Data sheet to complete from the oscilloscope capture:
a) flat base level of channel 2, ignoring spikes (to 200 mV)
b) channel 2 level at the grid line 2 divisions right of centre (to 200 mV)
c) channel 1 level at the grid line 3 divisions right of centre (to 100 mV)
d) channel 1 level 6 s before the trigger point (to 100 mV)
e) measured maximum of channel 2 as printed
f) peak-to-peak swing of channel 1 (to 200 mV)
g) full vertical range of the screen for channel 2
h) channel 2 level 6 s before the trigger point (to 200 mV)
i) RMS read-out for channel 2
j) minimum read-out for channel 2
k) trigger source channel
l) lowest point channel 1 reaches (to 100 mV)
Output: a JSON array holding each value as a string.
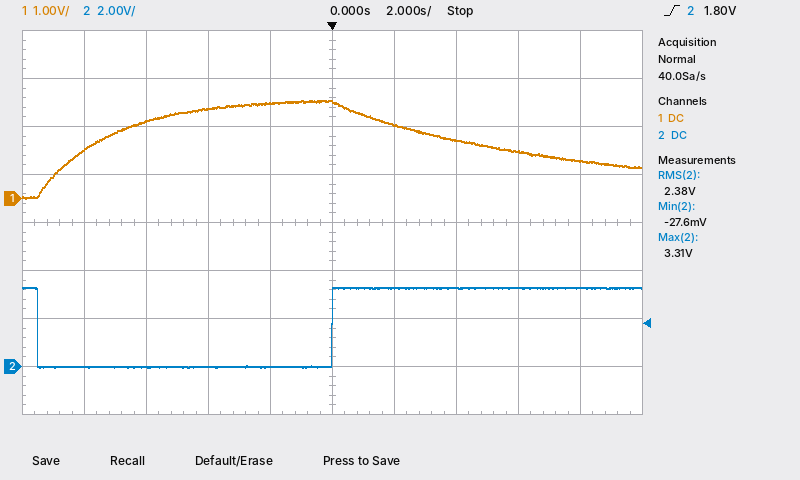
["0.0 V", "3.2 V", "1.0 V", "1.6 V", "3.31 V", "2.0 V", "16 V", "0.0 V", "2.38 V", "-27.6 mV", "channel 2", "0.0 V"]
